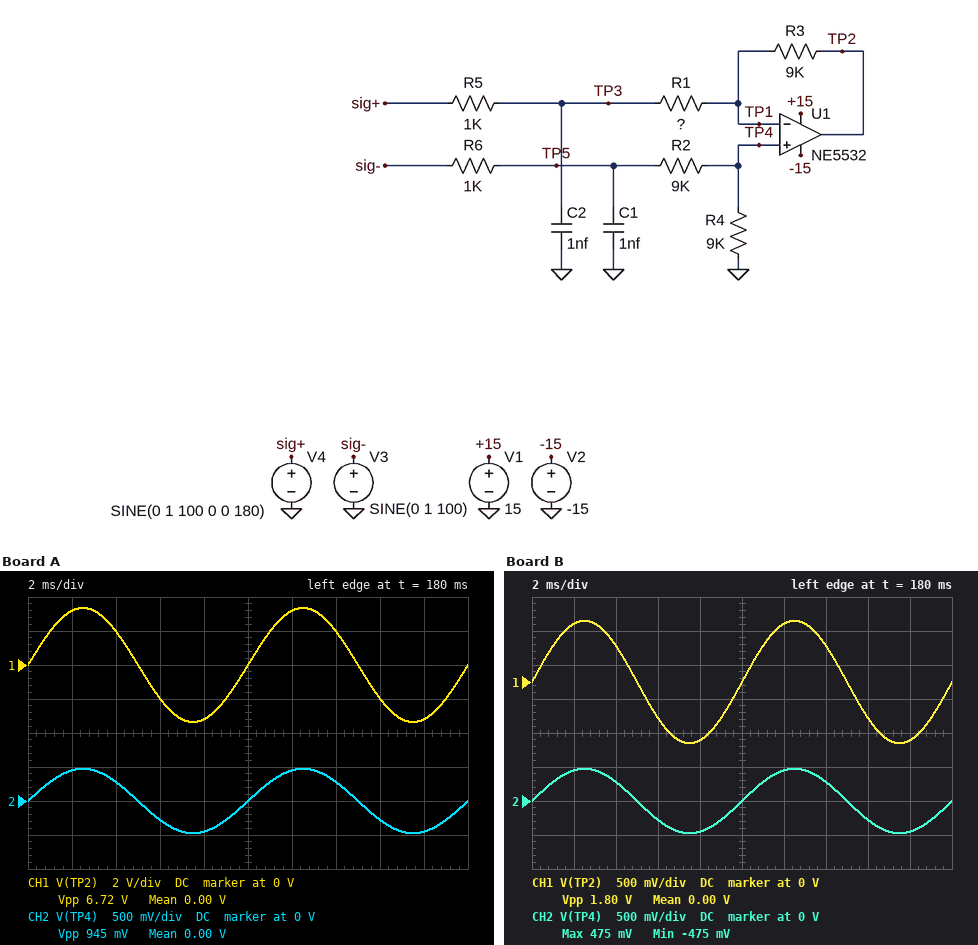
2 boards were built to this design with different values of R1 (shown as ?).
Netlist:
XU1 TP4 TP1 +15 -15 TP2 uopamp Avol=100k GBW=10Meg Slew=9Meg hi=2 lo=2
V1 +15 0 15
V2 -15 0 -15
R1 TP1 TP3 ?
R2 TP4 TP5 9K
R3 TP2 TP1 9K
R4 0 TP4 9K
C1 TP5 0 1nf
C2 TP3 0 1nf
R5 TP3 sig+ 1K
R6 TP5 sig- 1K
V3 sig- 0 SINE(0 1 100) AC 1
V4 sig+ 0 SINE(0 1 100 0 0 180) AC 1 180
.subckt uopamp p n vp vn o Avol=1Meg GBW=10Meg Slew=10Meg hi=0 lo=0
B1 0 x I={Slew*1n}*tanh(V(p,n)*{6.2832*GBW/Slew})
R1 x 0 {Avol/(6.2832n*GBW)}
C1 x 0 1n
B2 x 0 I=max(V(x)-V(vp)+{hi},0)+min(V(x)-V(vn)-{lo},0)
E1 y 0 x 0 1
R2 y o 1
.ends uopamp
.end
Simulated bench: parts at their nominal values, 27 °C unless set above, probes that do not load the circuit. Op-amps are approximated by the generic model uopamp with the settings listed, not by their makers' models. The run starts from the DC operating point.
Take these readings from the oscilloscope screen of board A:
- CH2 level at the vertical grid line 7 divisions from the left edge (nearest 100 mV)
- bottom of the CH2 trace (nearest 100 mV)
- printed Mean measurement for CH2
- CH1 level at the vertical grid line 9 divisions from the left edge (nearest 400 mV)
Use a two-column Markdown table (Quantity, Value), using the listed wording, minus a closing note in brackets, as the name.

| Quantity | Value |
|---|---|
| CH2 level at the vertical grid line 7 divisions from the left edge | 300 mV |
| bottom of the CH2 trace | -500 mV |
| printed Mean measurement for CH2 | 0.00 V |
| CH1 level at the vertical grid line 9 divisions from the left edge | -3.2 V |
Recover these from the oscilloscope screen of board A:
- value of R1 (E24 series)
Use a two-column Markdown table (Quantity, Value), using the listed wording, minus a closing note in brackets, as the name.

| Quantity | Value |
|---|---|
| value of R1 | 3.6 kΩ |
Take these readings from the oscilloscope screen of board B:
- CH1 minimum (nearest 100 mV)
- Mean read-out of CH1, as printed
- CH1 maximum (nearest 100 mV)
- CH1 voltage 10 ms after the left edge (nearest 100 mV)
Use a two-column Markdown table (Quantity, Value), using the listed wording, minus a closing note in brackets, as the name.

| Quantity | Value |
|---|---|
| CH1 minimum | -900 mV |
| Mean read-out of CH1, as printed | 0.00 V |
| CH1 maximum | 900 mV |
| CH1 voltage 10 ms after the left edge | 0 V |
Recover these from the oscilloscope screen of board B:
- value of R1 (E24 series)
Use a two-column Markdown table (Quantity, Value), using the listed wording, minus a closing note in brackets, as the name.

| Quantity | Value |
|---|---|
| value of R1 | 30 kΩ |
